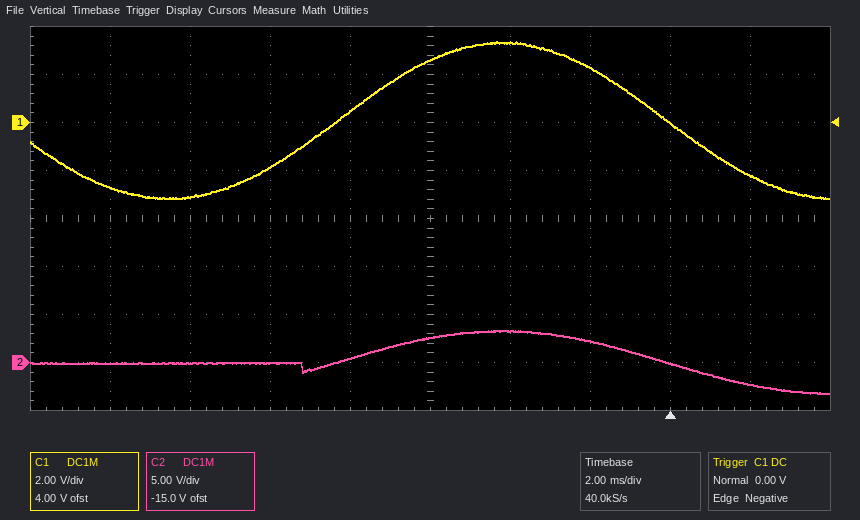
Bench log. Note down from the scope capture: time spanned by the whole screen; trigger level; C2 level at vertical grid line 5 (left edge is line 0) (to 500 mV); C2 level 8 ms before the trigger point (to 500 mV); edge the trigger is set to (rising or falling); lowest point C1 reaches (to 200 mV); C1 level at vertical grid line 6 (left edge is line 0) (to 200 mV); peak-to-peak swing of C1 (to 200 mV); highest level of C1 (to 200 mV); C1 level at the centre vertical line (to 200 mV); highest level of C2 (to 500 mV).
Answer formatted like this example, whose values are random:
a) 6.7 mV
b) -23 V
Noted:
a) 20 ms
b) 0.00 V
c) 2.5 V
d) 500 mV
e) falling
f) -3.2 V
g) 3.4 V
h) 6.6 V
i) 3.4 V
j) 2.6 V
k) 3.5 V
